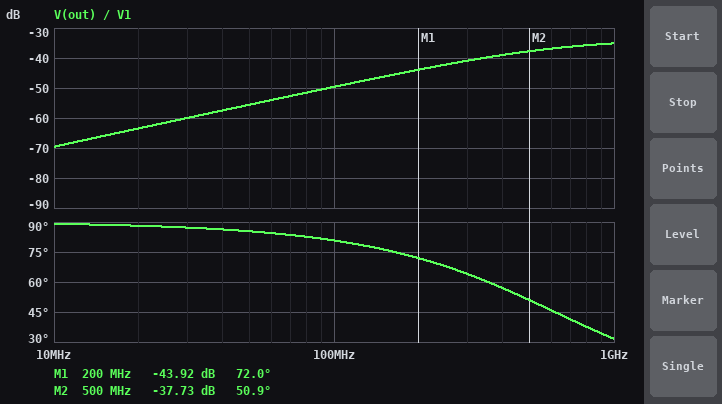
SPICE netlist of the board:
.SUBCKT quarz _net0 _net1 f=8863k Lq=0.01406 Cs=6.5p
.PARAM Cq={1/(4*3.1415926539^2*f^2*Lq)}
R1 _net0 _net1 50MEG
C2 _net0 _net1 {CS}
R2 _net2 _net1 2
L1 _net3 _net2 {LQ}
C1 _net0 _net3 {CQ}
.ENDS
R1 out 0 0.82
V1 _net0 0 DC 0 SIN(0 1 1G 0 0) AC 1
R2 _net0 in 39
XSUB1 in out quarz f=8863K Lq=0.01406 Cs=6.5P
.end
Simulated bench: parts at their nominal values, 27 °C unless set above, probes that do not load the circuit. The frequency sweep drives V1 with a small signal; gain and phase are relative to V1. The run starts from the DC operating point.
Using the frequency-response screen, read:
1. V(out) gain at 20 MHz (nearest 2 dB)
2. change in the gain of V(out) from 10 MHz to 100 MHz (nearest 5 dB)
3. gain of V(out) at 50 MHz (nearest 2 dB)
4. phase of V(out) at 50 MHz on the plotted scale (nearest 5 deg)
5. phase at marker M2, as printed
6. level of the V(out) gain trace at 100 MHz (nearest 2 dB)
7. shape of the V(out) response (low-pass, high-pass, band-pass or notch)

-64 dB
20 dB
-56 dB
85 deg
50.9 deg
-50 dB
high-pass
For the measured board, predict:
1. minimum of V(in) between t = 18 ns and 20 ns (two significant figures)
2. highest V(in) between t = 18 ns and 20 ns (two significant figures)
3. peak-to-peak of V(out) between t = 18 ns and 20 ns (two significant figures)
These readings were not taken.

-520 mV
520 mV
35 mV
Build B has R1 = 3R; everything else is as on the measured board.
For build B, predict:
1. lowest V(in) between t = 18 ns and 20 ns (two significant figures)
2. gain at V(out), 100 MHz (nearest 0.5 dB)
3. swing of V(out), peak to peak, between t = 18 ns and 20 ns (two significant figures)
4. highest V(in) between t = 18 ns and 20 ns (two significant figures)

-510 mV
-38.5 dB
120 mV
510 mV
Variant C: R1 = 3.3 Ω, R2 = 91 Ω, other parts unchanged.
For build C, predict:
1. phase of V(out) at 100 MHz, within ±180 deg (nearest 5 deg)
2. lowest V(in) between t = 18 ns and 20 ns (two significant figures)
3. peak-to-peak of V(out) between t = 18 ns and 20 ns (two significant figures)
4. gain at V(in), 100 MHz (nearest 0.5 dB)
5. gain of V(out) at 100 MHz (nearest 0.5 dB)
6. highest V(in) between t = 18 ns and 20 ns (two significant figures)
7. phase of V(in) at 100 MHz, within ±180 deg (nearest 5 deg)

70 deg
-250 mV
68 mV
-0.5 dB
-38.0 dB
250 mV
-20 deg
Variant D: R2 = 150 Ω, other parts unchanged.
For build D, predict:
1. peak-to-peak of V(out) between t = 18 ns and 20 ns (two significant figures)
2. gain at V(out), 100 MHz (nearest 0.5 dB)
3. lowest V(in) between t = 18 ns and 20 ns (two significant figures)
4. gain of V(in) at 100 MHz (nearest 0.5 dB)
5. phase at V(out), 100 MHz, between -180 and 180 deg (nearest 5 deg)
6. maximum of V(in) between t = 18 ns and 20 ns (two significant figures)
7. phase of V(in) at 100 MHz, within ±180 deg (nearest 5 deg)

11 mV
-51.0 dB
-160 mV
-1.5 dB
60 deg
160 mV
-30 deg
